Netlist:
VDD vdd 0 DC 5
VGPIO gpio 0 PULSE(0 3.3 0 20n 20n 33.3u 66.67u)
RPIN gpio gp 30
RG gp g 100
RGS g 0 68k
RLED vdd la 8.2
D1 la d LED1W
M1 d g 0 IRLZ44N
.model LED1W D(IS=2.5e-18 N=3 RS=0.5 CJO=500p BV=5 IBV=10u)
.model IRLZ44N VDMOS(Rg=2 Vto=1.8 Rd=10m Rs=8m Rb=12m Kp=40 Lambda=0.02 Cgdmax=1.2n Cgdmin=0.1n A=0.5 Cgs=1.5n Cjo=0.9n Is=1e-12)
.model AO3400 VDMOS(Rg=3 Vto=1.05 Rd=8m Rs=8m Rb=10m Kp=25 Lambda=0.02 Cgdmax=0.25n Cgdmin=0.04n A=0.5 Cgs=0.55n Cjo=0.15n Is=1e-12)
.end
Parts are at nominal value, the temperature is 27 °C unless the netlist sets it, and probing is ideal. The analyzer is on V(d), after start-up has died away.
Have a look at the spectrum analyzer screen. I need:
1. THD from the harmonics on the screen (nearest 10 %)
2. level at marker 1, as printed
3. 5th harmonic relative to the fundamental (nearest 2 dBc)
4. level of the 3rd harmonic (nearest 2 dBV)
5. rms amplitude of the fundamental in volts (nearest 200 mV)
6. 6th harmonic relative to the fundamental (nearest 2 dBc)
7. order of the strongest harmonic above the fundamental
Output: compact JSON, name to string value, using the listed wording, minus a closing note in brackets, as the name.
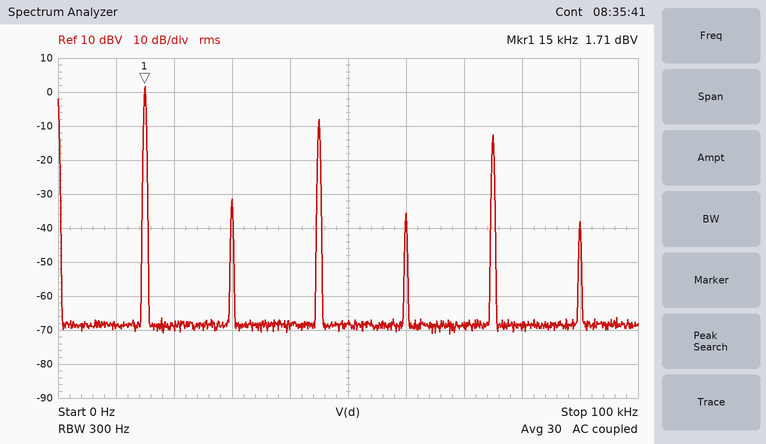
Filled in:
{"THD from the harmonics on the screen": "40 %", "level at marker 1, as printed": "1.71 dBV", "5th harmonic relative to the fundamental": "-14 dBc", "level of the 3rd harmonic": "-8 dBV", "rms amplitude of the fundamental in volts": "1.2 V", "6th harmonic relative to the fundamental": "-40 dBc", "order of the strongest harmonic above the fundamental": "3"}
